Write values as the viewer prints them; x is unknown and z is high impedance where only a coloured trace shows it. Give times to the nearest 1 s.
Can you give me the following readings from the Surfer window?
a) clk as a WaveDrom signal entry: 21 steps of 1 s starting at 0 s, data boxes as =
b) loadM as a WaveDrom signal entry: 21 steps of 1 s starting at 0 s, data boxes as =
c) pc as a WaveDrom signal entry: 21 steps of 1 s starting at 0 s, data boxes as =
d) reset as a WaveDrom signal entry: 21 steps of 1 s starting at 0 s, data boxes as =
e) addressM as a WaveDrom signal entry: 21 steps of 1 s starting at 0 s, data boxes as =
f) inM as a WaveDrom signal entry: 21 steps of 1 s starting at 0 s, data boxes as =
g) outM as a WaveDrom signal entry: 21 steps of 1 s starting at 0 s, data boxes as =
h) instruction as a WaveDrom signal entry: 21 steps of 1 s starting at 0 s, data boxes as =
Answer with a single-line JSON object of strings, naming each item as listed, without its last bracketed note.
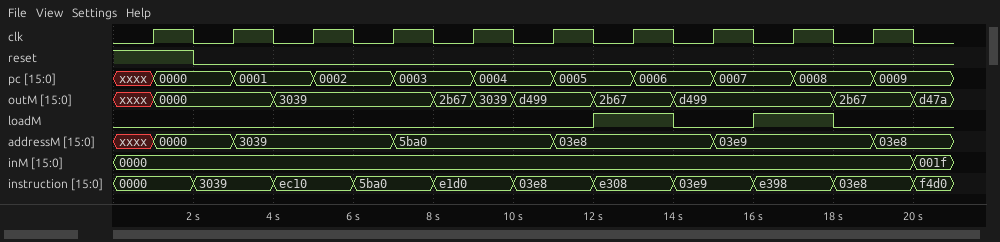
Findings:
{"clk as a WaveDrom signal entry: 21 steps of 1 s starting at 0 s, data boxes as =": "{name: 'clk', wave: '010101010101010101010'}", "loadM as a WaveDrom signal entry: 21 steps of 1 s starting at 0 s, data boxes as =": "{name: 'loadM', wave: '0...........1.0.1.0..'}", "pc as a WaveDrom signal entry: 21 steps of 1 s starting at 0 s, data boxes as =": "{name: 'pc', wave: 'x=.=.=.=.=.=.=.=.=.=.', data: '0000 0001 0002 0003 0004 0005 0006 0007 0008 0009'}", "reset as a WaveDrom signal entry: 21 steps of 1 s starting at 0 s, data boxes as =": "{name: 'reset', wave: '1.0..................'}", "addressM as a WaveDrom signal entry: 21 steps of 1 s starting at 0 s, data boxes as =": "{name: 'addressM', wave: 'x=.=...=...=...=...=.', data: '0000 3039 5ba0 03e8 03e9 03e8'}", "inM as a WaveDrom signal entry: 21 steps of 1 s starting at 0 s, data boxes as =": "{name: 'inM', wave: '=...................=', data: '0000 001f'}", "outM as a WaveDrom signal entry: 21 steps of 1 s starting at 0 s, data boxes as =": "{name: 'outM', wave: 'x=..=...===.=.=...=.=', data: '0000 3039 2b67 3039 d499 2b67 d499 2b67 d47a'}", "instruction as a WaveDrom signal entry: 21 steps of 1 s starting at 0 s, data boxes as =": "{name: 'instruction', wave: '=.=.=.=.=.=.=.=.=.=.=', data: '0000 3039 ec10 5ba0 e1d0 03e8 e308 03e9 e398 03e8 f4d0'}"}
